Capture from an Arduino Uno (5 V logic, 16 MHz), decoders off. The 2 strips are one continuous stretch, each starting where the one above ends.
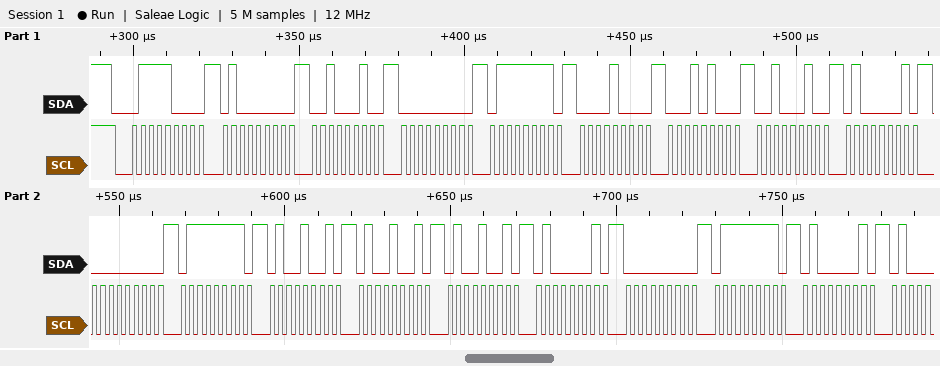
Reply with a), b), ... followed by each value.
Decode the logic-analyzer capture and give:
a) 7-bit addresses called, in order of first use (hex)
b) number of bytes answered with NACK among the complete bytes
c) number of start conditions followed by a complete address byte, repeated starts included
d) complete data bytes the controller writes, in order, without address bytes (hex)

a) 0x3C
b) 0
c) 1
d) 40 22 00 7F 08 14 22 41 00 7F 49 49 49 41 00 7F 41
